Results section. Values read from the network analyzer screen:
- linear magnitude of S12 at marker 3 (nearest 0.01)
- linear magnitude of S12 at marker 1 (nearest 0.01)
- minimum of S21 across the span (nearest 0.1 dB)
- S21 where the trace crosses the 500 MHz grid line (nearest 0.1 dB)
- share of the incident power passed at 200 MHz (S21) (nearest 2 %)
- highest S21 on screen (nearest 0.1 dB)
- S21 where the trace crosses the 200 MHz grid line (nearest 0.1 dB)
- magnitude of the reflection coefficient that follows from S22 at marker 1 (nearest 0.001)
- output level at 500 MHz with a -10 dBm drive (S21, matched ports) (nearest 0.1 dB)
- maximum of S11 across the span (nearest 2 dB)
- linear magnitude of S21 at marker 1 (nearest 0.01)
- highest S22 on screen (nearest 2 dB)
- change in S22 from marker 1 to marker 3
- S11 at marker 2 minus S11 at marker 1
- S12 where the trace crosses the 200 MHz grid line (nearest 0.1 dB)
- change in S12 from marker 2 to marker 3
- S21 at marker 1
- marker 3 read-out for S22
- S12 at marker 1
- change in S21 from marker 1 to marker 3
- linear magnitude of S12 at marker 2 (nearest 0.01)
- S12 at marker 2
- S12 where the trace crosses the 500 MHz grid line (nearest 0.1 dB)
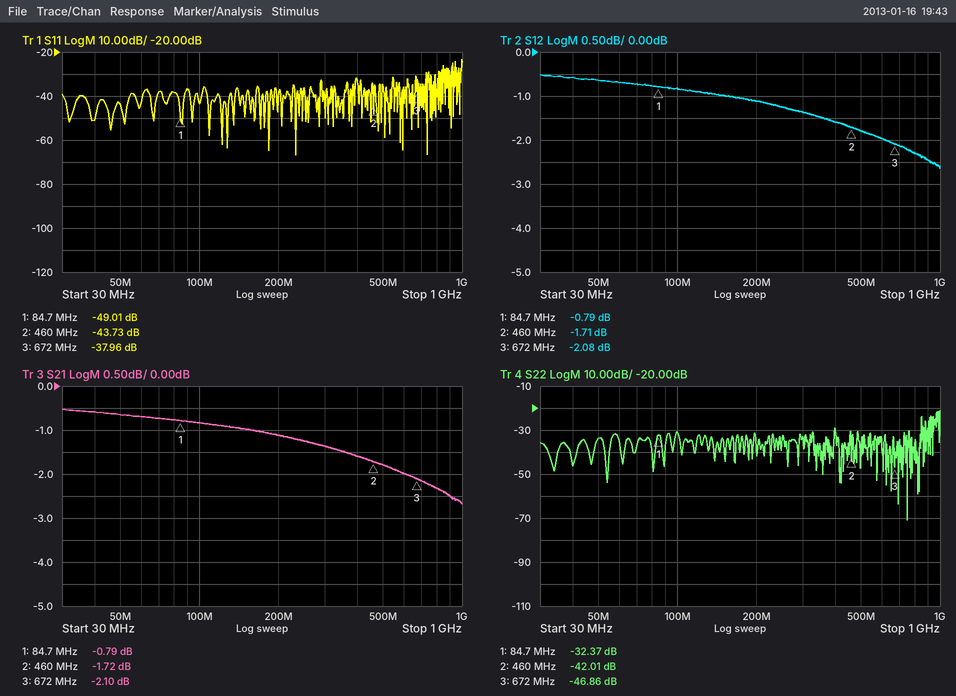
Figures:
0.79
0.91
-2.7 dB
-1.8 dB
78 %
-0.5 dB
-1.1 dB
0.024
-11.8 dBm
-24 dB
0.91
-22 dB
-14.49 dB
5.28 dB
-1.1 dB
-0.37 dB
-0.79 dB
-46.86 dB
-0.79 dB
-1.31 dB
0.82
-1.71 dB
-1.8 dB
